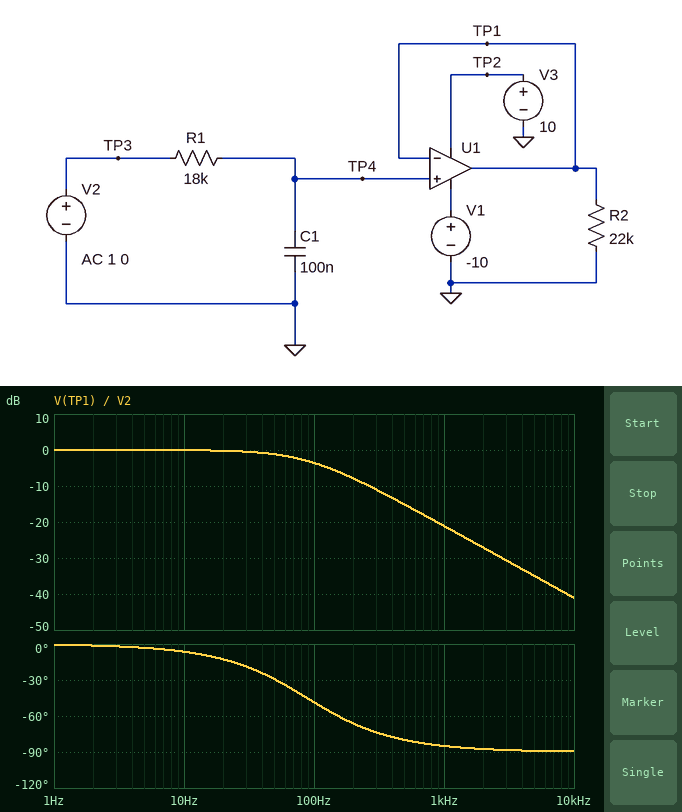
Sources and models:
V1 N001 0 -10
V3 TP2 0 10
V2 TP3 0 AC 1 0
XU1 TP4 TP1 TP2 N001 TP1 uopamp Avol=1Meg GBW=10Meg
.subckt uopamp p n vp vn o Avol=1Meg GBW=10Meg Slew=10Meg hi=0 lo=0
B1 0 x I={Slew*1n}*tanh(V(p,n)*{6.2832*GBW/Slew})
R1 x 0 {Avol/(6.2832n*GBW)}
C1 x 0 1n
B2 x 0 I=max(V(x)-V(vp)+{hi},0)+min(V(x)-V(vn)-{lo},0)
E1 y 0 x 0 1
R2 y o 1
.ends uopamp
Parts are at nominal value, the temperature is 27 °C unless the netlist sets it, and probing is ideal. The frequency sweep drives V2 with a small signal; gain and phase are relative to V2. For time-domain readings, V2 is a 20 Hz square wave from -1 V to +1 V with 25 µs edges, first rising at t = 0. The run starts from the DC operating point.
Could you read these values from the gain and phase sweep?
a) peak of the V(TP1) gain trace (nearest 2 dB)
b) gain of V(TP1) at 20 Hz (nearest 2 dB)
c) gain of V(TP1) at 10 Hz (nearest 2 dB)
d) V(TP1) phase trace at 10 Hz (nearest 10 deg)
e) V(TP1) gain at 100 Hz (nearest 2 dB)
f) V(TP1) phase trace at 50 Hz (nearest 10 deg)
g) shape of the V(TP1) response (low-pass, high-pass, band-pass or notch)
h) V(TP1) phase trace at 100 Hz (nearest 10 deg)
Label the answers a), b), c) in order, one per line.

a) 0 dB
b) 0 dB
c) 0 dB
d) -10 deg
e) -4 dB
f) -30 deg
g) low-pass
h) -50 deg
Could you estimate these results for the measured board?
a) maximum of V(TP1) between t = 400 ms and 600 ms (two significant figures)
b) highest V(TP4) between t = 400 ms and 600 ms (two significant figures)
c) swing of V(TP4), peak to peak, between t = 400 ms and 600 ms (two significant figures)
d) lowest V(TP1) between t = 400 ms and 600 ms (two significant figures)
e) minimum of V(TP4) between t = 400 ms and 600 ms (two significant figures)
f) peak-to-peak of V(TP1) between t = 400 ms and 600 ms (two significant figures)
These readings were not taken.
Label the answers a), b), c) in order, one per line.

a) 1.0 V
b) 1.0 V
c) 2.0 V
d) -1.0 V
e) -1.0 V
f) 2.0 V
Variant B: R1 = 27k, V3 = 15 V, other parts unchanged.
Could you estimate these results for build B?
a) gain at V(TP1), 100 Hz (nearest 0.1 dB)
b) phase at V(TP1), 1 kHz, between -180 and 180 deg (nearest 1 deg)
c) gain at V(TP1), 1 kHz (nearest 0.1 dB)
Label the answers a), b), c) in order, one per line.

a) -5.9 dB
b) -87 deg
c) -24.6 dB
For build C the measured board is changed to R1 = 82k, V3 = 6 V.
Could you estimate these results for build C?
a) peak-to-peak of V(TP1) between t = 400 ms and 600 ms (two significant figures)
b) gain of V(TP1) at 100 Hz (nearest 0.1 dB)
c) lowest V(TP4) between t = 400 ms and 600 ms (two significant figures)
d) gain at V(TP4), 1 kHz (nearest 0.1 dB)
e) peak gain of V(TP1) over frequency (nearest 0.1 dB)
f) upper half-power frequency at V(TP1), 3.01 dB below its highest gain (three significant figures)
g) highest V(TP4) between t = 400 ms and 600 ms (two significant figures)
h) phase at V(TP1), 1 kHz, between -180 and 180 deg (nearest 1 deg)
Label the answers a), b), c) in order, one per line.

a) 1.8 V
b) -14.4 dB
c) -910 mV
d) -34.2 dB
e) 0 dB
f) 19.4 Hz
g) 910 mV
h) -89 deg
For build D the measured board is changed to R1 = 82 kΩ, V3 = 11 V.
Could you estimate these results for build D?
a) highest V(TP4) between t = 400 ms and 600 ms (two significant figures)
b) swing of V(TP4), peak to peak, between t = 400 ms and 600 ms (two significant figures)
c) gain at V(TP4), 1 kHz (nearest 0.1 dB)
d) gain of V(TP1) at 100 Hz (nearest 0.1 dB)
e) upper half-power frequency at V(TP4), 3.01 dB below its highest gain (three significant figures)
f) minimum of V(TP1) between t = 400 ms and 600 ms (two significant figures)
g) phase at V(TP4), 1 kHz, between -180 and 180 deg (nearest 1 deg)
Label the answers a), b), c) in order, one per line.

a) 910 mV
b) 1.8 V
c) -34.2 dB
d) -14.4 dB
e) 19.4 Hz
f) -910 mV
g) -89 deg
